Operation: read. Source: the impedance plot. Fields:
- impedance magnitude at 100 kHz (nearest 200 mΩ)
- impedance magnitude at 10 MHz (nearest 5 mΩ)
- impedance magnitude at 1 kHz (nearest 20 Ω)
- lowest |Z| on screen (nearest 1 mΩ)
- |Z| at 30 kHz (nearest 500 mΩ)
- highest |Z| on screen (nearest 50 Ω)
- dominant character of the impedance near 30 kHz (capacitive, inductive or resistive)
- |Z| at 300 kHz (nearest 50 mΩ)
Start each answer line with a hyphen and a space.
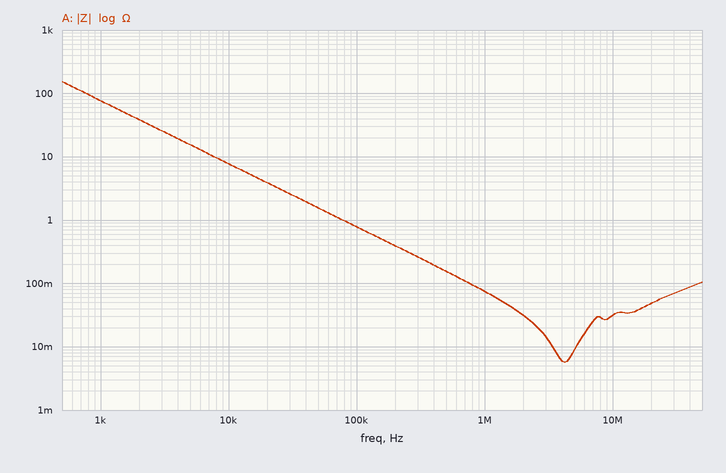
- 800 mΩ
- 30 mΩ
- 80 Ω
- 6 mΩ
- 2.5 Ω
- 150 Ω
- capacitive
- 250 mΩ
